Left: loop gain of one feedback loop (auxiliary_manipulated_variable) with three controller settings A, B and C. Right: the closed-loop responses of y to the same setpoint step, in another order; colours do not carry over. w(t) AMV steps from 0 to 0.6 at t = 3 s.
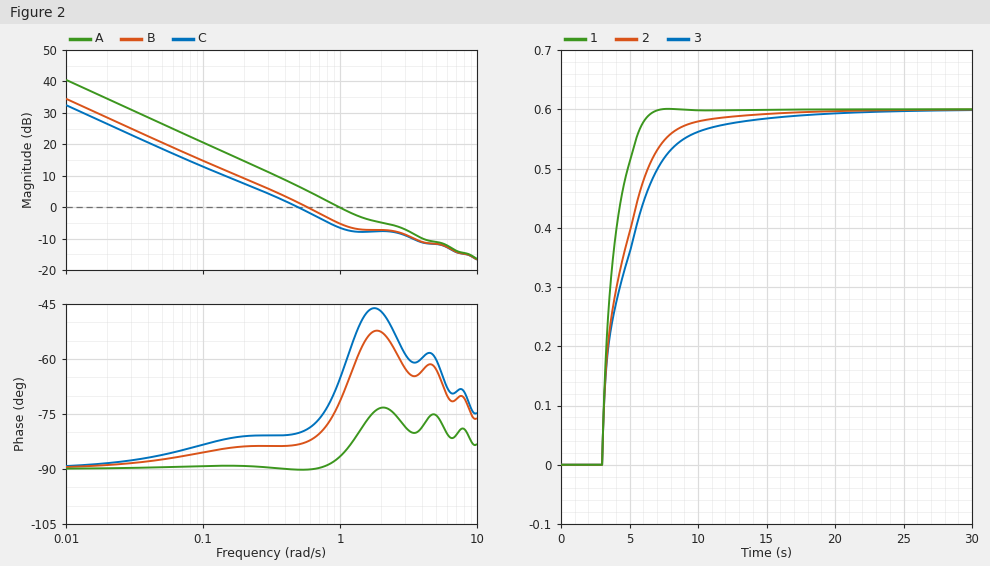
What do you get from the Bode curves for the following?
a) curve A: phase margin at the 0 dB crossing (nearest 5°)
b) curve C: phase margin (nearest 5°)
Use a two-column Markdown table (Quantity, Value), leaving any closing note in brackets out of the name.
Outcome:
| Quantity | Value |
|---|---|
| curve A: phase margin at the 0 dB crossing | 95° |
| curve C: phase margin | 100° |
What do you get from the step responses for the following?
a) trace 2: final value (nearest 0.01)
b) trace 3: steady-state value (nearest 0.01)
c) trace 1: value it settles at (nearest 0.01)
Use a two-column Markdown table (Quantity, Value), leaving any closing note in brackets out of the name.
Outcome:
| Quantity | Value |
|---|---|
| trace 2: final value | 0.60 |
| trace 3: steady-state value | 0.60 |
| trace 1: value it settles at | 0.60 |
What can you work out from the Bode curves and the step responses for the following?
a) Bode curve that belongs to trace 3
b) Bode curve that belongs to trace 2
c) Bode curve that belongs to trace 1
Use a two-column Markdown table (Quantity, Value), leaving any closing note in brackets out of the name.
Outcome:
| Quantity | Value |
|---|---|
| Bode curve that belongs to trace 3 | C |
| Bode curve that belongs to trace 2 | B |
| Bode curve that belongs to trace 1 | A |
